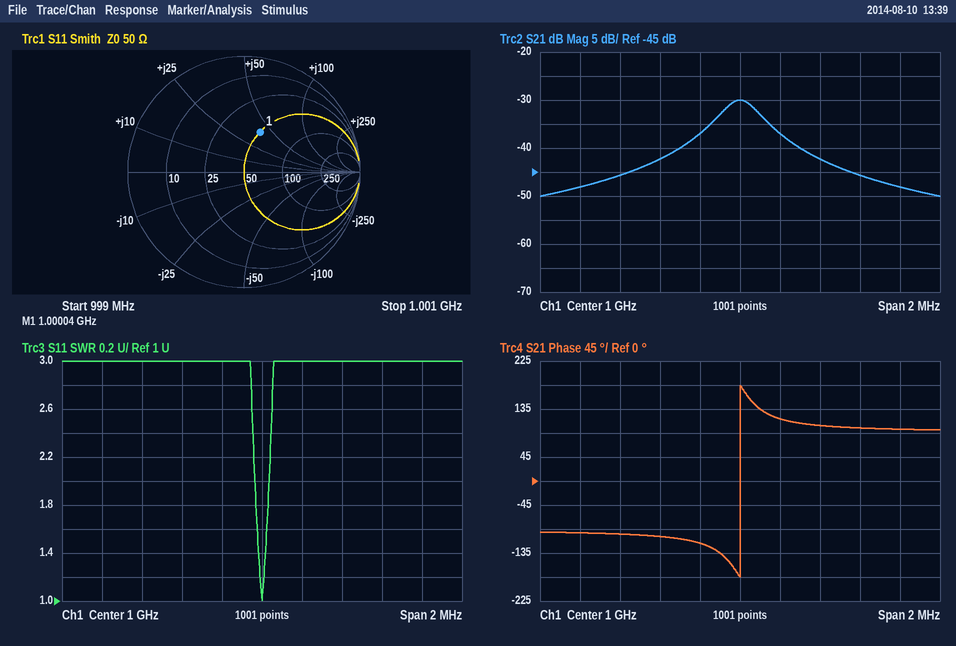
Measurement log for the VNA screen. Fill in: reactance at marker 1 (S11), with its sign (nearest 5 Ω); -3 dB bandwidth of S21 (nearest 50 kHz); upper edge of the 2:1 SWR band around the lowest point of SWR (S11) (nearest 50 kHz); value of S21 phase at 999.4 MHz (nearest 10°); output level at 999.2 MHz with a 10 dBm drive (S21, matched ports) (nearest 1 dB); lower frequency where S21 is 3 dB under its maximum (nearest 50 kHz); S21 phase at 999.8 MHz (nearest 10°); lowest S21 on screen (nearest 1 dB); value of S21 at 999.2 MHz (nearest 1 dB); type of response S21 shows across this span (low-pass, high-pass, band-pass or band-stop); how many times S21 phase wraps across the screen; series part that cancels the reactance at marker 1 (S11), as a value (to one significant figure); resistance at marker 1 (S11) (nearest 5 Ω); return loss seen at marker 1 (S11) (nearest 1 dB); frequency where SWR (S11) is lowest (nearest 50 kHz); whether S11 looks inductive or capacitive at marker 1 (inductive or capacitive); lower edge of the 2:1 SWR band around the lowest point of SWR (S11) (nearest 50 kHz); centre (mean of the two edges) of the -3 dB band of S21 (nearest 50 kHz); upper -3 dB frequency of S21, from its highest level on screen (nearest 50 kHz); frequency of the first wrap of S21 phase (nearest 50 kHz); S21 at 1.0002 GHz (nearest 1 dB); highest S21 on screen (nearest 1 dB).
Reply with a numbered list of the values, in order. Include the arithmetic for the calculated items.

1. +40 Ω
2. 1.00010 GHz − 999.90 MHz = 200 kHz
3. 1.00005 GHz
4. -100°
5. 10 dBm + (-48 dB) = -38 dBm
6. 999.90 MHz
7. -120°
8. -50 dB
9. -48 dB
10. band-pass
11. 1
12. C = 1/(2π × 1.00004 GHz × 40 Ω) ≈ 4 pF
13. 50 Ω
14. 9 dB
15. 1.00000 GHz
16. inductive
17. 999.95 MHz
18. 1.00000 GHz
19. 1.00010 GHz
20. 1.00000 GHz
21. -37 dB
22. -30 dB
